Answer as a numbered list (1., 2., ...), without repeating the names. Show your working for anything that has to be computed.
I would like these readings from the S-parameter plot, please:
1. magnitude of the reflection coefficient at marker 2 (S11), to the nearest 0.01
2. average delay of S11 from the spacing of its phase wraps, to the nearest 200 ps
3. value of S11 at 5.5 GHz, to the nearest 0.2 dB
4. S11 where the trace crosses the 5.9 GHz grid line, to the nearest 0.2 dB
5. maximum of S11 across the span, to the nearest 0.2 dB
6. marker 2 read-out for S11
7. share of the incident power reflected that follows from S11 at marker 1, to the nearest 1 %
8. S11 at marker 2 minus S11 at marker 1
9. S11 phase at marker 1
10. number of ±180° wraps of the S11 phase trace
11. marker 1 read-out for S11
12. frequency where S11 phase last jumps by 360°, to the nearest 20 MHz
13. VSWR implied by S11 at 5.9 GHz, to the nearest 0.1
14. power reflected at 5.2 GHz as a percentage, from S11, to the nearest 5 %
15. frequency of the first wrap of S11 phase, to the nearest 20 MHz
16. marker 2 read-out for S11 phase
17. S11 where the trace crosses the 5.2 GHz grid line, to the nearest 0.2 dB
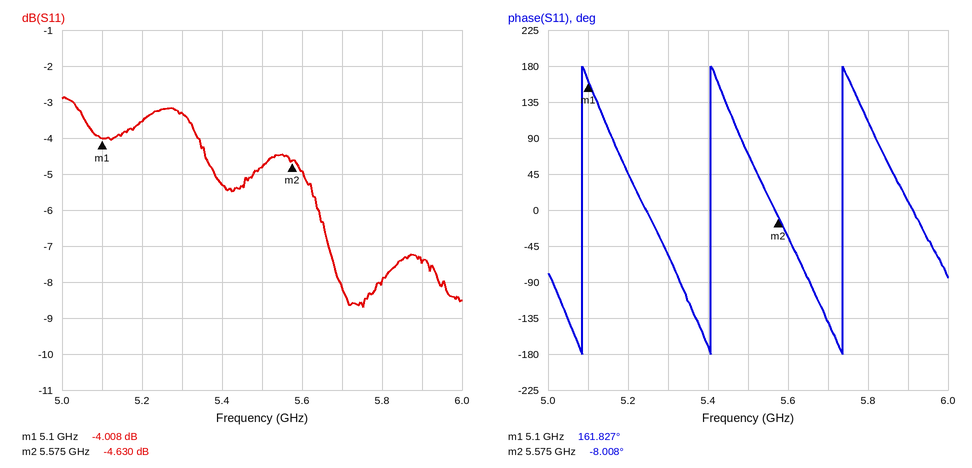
1. 10^(-4.63/20) ≈ 0.59
2. 2 cycles / (5.74 GHz − 5.08 GHz) ≈ 3.0 ns
3. -4.8 dB
4. -7.4 dB
5. -2.8 dB
6. -4.630 dB
7. 10^(-4.008/10) ≈ 40 %
8. -4.63 − (-4.008) = -0.622 dB
9. 161.827°
10. 3
11. -4.008 dB
12. 5.74 GHz
13. |Γ| = 10^(-7.4/20) = 0.4266; VSWR = (1 + 0.4266)/(1 − 0.4266) ≈ 2.5
14. 10^(-3.6/10) ≈ 43.7 %, so 45 % to the nearest 5 %
15. 5.08 GHz
16. -8.008°
17. -3.6 dB
